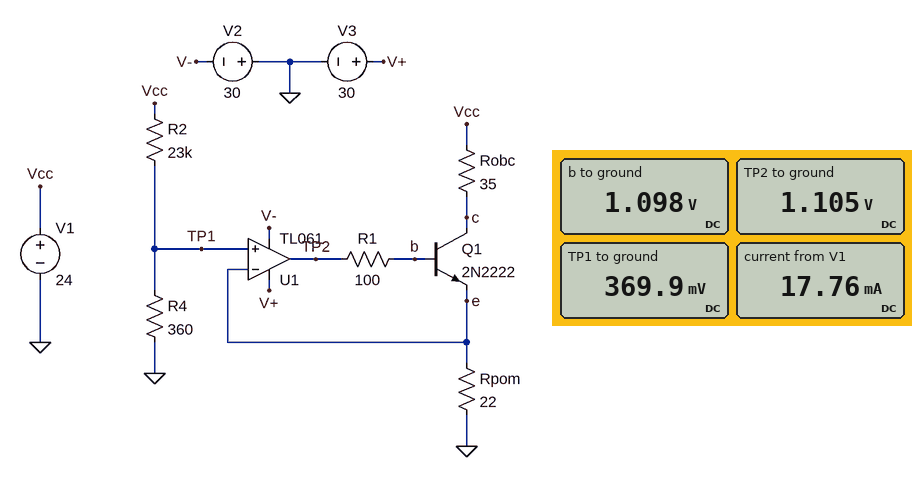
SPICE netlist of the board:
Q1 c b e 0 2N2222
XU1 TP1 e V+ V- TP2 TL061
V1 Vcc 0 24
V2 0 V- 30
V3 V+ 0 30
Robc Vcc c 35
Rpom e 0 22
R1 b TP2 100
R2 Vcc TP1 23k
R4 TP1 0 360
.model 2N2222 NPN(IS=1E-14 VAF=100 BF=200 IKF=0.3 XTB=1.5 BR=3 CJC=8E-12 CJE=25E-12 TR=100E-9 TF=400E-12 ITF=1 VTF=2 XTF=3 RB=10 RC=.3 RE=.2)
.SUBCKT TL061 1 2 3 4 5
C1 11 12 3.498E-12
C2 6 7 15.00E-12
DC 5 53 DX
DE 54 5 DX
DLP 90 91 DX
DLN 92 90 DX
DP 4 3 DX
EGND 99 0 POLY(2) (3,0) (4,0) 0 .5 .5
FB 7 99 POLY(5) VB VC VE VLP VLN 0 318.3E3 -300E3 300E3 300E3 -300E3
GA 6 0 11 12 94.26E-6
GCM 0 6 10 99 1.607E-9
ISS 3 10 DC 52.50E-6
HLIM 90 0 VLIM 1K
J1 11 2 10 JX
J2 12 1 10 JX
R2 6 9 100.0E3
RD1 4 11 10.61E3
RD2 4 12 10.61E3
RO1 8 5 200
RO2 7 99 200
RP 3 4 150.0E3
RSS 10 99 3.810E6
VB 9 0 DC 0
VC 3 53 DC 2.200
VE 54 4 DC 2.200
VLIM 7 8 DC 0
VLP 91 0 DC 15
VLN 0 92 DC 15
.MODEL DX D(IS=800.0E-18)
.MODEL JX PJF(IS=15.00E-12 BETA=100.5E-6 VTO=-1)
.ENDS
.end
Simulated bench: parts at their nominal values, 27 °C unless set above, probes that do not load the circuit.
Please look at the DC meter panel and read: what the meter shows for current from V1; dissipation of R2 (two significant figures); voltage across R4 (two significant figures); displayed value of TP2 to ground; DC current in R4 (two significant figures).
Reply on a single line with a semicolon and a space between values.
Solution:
17.76 mA; 24 mW; 370 mV; 1.105 V; 1.0 mA
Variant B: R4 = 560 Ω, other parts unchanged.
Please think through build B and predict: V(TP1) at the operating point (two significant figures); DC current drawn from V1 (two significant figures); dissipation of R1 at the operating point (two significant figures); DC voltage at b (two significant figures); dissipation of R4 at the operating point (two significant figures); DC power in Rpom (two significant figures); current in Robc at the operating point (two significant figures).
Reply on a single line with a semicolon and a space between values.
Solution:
570 mV; 27 mA; 1.3 µW; 1.3 V; 580 µW; 15 mW; 26 mA
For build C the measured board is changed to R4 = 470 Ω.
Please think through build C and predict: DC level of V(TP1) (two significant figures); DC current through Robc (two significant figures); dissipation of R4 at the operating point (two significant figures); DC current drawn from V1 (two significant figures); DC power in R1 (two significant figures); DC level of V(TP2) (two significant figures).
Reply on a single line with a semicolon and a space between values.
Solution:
480 mV; 22 mA; 490 µW; 23 mA; 890 nW; 1.2 V
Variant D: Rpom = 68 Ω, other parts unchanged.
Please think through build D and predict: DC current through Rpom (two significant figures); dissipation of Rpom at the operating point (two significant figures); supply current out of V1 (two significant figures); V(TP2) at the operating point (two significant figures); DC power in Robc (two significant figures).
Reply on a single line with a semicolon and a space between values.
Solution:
5.4 mA; 2.0 mW; 6.4 mA; 1.1 V; 1.0 mW
